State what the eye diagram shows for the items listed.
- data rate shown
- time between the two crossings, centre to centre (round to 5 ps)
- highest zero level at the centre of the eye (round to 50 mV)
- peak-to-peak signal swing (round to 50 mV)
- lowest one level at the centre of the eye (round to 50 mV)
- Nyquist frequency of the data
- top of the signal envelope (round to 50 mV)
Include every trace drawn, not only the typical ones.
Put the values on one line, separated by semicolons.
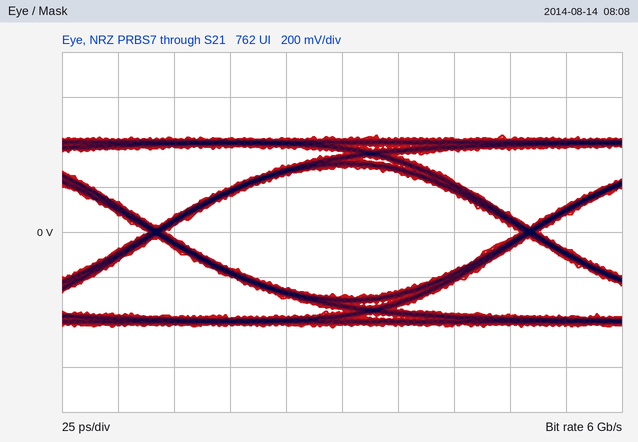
6 Gb/s; 165 ps; -300 mV; 850 mV; 300 mV; 3 GHz; 450 mV
